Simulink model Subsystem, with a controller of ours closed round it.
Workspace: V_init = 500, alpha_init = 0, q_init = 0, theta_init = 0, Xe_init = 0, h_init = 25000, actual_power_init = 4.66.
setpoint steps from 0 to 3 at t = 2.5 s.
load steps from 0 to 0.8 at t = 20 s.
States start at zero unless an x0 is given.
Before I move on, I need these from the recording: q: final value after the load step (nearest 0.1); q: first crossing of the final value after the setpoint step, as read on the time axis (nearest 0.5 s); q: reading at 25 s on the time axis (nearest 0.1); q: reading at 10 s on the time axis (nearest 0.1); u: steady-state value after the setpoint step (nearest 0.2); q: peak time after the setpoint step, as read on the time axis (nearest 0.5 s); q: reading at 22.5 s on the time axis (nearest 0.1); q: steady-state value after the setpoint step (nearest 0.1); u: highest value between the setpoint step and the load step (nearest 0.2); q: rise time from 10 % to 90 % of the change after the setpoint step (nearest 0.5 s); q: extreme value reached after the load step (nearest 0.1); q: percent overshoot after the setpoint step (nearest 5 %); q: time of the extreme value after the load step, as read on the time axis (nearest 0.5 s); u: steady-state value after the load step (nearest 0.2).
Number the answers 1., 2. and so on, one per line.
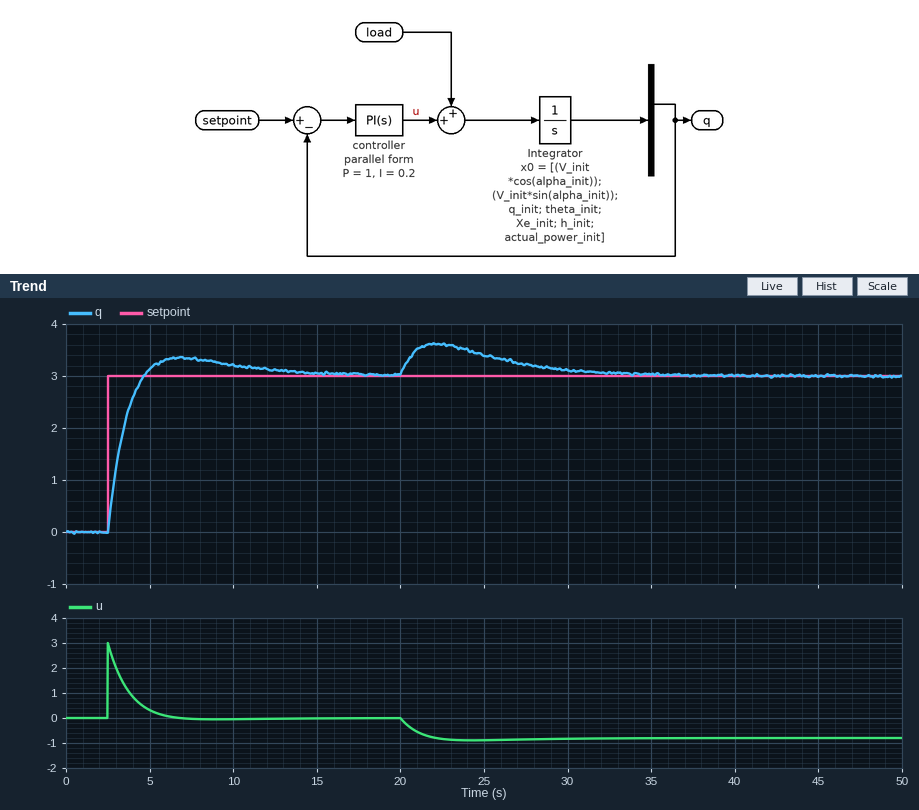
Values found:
1. 3.0
2. 4.5 s
3. 3.4
4. 3.2
5. 0.0
6. 7.0 s
7. 3.6
8. 3.0
9. 3.0
10. 1.5 s
11. 3.6
12. 10 %
13. 22.0 s
14. -0.8
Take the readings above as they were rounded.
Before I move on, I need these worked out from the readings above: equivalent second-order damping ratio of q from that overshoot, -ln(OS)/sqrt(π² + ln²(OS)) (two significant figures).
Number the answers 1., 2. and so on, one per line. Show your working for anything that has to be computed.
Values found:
1. ln(0.1) = -2.303; 2.303 / sqrt(9.870 + 5.302) = 0.59
